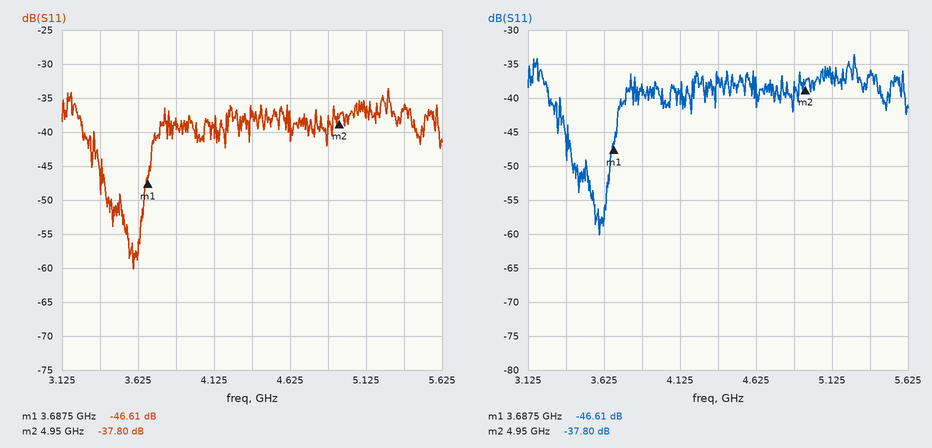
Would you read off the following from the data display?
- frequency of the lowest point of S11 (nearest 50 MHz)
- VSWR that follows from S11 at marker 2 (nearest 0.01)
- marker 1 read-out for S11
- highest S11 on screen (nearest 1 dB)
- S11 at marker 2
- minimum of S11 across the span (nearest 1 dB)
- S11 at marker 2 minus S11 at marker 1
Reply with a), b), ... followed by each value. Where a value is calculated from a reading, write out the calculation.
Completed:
a) 3.60 GHz
b) (1 + 0.0129)/(1 − 0.0129) ≈ 1.03
c) -46.61 dB
d) -34 dB
e) -37.80 dB
f) -60 dB
g) -37.8 − (-46.61) = 8.81 dB
